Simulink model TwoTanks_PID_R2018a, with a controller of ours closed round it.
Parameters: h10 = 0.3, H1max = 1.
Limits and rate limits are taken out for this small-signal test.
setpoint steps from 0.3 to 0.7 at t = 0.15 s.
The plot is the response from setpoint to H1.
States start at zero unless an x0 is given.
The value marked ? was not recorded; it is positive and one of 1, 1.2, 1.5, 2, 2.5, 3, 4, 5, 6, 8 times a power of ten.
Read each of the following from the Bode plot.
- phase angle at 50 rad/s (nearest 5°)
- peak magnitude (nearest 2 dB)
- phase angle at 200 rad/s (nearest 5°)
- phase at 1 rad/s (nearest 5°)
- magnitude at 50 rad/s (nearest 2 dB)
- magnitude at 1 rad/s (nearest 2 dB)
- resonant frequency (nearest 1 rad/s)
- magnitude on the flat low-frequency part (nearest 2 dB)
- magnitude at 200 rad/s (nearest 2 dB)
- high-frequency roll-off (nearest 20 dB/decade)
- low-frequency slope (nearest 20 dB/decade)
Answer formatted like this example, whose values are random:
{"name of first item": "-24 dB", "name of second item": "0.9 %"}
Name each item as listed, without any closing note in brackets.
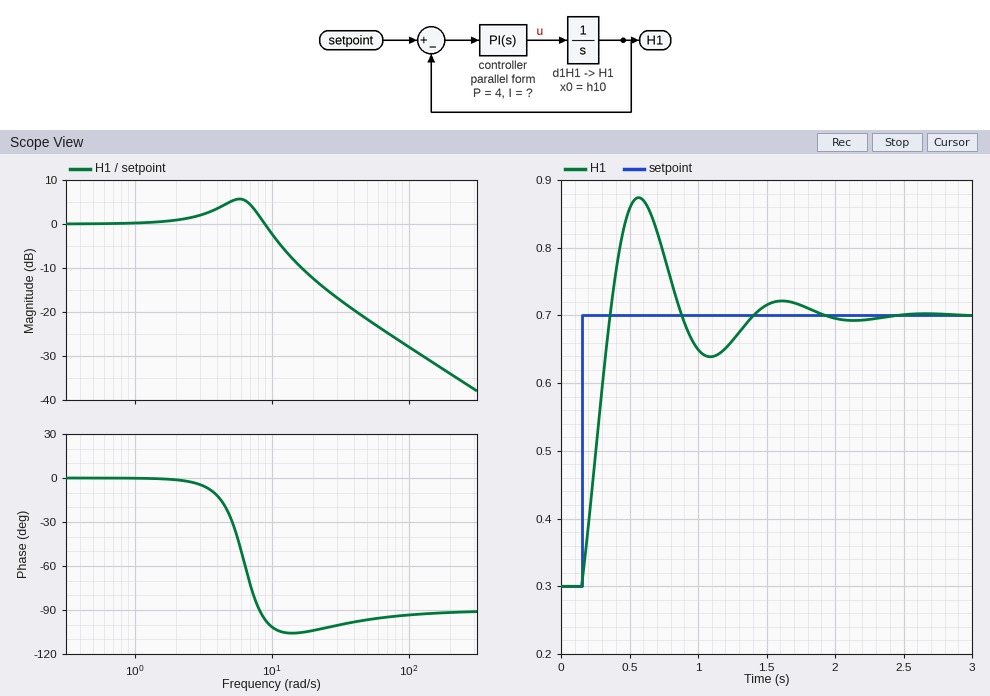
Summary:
{"phase angle at 50 rad/s": "-95°", "peak magnitude": "6 dB", "phase angle at 200 rad/s": "-90°", "phase at 1 rad/s": "0°", "magnitude at 50 rad/s": "-22 dB", "magnitude at 1 rad/s": "0 dB", "resonant frequency": "6 rad/s", "magnitude on the flat low-frequency part": "0 dB", "magnitude at 200 rad/s": "-34 dB", "high-frequency roll-off": "-20 dB/decade", "low-frequency slope": "0 dB/decade"}
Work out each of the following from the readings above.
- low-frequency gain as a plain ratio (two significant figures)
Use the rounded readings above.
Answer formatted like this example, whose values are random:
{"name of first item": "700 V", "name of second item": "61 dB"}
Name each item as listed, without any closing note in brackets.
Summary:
{"low-frequency gain as a plain ratio": "1.0"}
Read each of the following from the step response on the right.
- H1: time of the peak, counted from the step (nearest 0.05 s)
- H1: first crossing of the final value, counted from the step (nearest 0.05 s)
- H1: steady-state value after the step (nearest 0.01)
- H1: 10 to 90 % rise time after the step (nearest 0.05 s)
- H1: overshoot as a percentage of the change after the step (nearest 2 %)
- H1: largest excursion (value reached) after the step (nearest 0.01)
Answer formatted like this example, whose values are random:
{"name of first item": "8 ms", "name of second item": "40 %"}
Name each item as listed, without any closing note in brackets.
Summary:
{"H1: time of the peak, counted from the step": "0.40 s", "H1: first crossing of the final value, counted from the step": "0.20 s", "H1: steady-state value after the step": "0.70", "H1: 10 to 90 % rise time after the step": "0.15 s", "H1: overshoot as a percentage of the change after the step": "44 %", "H1: largest excursion (value reached) after the step": "0.87"}
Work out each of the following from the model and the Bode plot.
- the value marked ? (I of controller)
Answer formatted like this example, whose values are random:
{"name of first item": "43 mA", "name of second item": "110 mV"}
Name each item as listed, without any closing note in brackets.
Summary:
{"the value marked ?": "40"}
